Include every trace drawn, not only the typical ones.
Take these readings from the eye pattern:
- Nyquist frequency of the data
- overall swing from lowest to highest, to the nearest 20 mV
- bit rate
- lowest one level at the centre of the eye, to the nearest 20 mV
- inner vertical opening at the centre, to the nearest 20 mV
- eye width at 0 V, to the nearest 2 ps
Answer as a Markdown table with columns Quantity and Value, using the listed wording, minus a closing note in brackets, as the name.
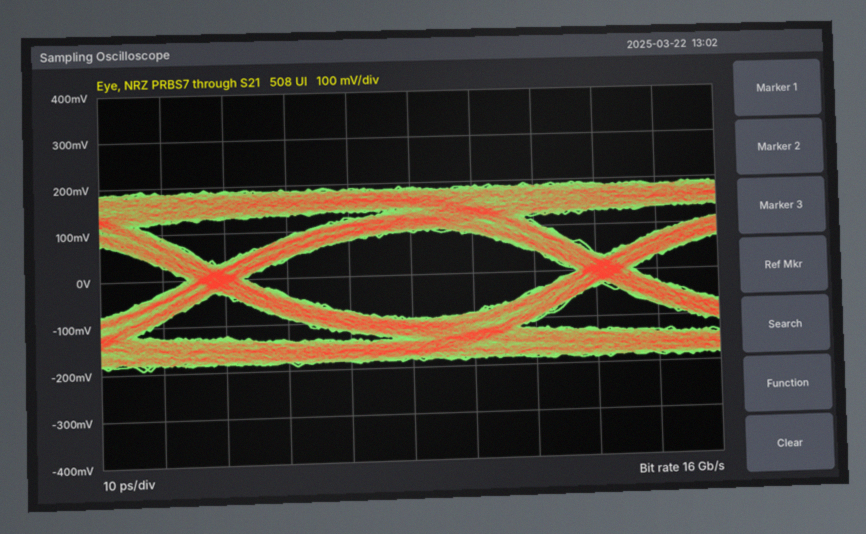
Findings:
| Quantity | Value |
|---|---|
| Nyquist frequency of the data | 8 GHz |
| overall swing from lowest to highest, to the nearest 20 mV | 380 mV |
| bit rate | 16 Gb/s |
| lowest one level at the centre of the eye, to the nearest 20 mV | 100 mV |
| inner vertical opening at the centre, to the nearest 20 mV | 180 mV |
| eye width at 0 V, to the nearest 2 ps | 54 ps |
